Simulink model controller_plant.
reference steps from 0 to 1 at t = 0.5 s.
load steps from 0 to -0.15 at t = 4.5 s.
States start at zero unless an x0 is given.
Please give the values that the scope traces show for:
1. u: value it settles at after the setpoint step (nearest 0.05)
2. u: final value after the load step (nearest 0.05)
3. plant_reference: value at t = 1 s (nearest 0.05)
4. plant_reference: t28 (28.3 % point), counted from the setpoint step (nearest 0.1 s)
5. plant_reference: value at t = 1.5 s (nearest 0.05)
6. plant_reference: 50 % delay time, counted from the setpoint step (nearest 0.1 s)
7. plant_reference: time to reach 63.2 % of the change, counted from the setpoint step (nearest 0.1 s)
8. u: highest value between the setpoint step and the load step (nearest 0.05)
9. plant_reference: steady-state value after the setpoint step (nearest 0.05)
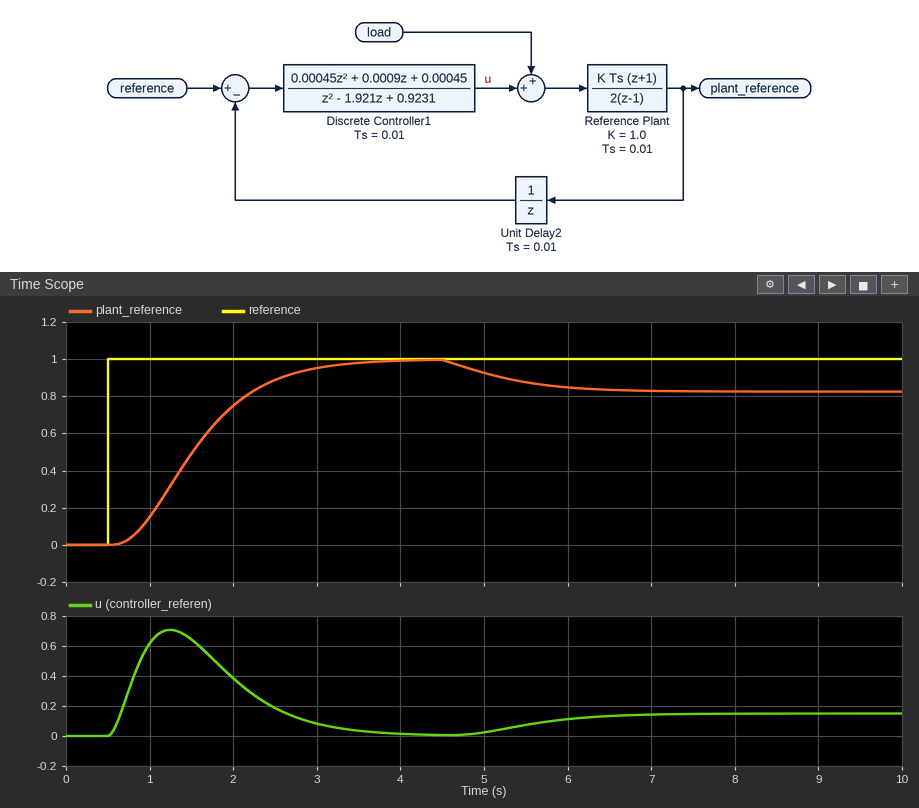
0.00
0.15
0.15
0.7 s
0.50
1.0 s
1.2 s
0.70
1.00
